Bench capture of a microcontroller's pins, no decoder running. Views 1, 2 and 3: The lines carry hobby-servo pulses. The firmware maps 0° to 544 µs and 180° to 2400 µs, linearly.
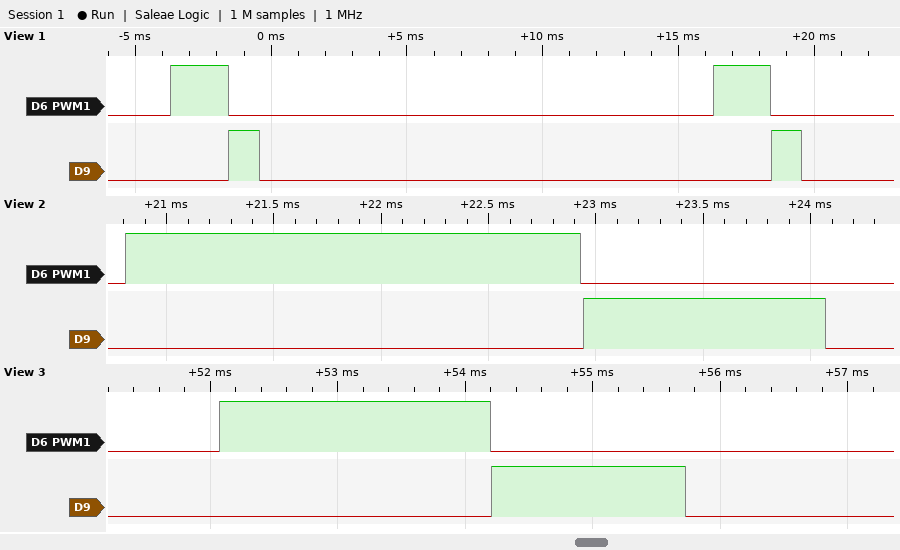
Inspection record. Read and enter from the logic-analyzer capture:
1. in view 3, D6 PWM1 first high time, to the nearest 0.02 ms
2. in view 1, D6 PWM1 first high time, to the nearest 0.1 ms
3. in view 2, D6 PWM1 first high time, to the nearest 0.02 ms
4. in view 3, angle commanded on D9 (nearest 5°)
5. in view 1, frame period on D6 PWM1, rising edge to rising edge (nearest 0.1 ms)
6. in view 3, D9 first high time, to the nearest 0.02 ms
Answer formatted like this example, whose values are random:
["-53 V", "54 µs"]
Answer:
["2.12 ms", "2.1 ms", "2.12 ms", "95°", "20.0 ms", "1.52 ms"]
